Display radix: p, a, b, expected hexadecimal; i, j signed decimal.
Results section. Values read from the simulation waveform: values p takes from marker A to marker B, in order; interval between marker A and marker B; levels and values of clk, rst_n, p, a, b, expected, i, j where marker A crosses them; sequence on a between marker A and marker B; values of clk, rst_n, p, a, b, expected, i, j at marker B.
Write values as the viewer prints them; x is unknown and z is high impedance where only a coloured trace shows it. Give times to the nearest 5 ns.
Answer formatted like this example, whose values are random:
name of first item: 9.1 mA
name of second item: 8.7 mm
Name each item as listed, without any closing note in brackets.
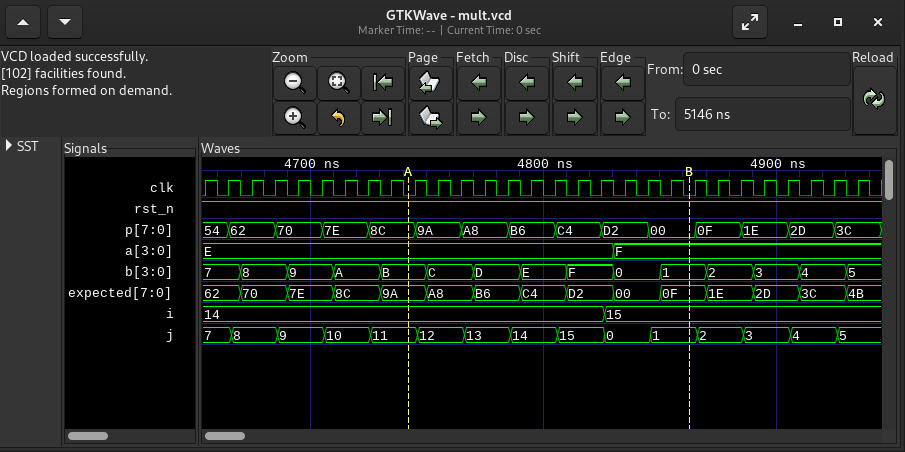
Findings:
values p takes from marker A to marker B, in order: 8C, 9A, A8, B6, C4, D2, 00
interval between marker A and marker B: 120 ns
levels and values of clk, rst_n, p, a, b, expected, i, j where marker A crosses them: clk=0, rst_n=1, p=8C, a=E, b=B, expected=9A, i=14, j=11
sequence on a between marker A and marker B: E, F
values of clk, rst_n, p, a, b, expected, i, j at marker B: clk=0, rst_n=1, p=00, a=F, b=1, expected=0F, i=15, j=1
